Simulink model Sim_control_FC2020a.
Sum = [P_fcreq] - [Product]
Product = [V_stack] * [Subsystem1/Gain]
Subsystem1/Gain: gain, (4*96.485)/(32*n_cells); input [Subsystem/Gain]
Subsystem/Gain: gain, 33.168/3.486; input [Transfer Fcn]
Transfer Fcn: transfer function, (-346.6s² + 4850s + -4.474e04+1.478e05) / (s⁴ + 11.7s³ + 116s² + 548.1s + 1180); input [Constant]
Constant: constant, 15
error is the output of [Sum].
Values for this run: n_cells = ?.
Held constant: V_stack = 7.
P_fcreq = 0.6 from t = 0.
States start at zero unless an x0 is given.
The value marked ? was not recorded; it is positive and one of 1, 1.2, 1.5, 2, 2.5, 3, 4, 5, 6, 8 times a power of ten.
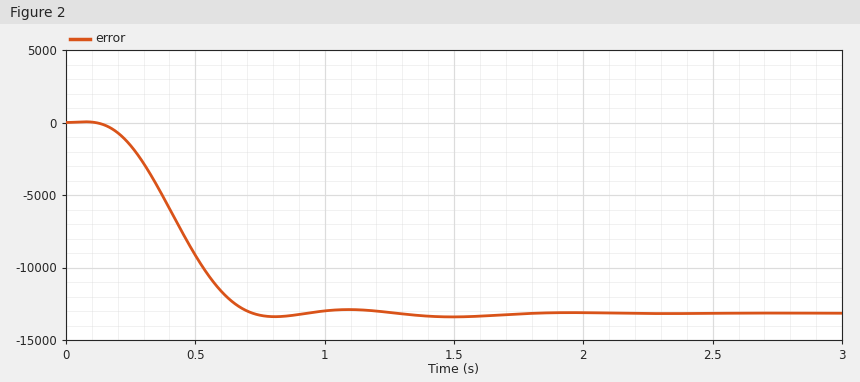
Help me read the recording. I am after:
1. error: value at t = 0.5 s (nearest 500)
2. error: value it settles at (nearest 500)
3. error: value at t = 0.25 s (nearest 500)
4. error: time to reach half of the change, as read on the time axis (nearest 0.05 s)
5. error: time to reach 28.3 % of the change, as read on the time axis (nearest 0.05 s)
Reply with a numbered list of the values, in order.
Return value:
1. -9000
2. -13000
3. -1500
4. 0.40 s
5. 0.35 s
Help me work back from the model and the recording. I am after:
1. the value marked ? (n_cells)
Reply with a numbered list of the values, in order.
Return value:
1. 80
